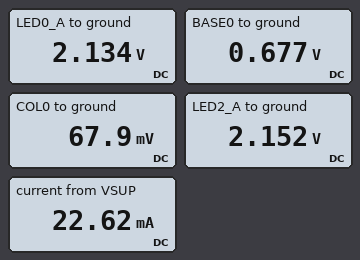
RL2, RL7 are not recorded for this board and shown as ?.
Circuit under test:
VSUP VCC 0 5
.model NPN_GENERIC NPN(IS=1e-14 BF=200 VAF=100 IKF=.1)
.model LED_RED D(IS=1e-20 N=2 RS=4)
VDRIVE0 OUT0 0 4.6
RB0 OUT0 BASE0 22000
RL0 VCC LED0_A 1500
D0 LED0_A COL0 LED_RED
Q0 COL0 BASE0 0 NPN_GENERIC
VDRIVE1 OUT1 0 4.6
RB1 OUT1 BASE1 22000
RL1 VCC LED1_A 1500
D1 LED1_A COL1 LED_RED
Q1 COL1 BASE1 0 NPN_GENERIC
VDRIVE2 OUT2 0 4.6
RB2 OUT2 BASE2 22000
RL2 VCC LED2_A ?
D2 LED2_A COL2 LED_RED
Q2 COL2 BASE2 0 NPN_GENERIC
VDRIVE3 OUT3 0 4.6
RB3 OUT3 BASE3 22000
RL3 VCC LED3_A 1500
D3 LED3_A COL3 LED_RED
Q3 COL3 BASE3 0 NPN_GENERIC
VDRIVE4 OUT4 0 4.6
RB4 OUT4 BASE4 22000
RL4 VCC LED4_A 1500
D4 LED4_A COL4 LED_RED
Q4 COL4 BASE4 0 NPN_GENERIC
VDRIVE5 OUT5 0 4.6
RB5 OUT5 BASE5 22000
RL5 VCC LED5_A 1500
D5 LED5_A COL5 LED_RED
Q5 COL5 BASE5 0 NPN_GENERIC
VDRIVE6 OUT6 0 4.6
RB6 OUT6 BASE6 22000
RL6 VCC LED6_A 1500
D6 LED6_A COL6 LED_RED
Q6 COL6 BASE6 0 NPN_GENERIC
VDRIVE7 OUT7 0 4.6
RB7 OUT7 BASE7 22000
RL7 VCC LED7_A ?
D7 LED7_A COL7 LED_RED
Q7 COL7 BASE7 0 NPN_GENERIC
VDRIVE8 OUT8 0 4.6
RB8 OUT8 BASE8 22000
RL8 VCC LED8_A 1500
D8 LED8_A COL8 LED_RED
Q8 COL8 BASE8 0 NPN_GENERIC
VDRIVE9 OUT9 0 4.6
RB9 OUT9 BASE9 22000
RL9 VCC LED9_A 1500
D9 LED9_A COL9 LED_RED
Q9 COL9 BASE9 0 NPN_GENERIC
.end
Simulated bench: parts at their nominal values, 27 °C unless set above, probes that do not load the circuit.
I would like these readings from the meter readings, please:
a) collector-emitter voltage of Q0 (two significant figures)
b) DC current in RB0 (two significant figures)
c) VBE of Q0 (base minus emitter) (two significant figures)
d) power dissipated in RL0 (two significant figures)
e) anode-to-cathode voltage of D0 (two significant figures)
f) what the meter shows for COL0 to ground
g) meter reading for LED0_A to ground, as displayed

68 mV
180 µA
680 mV
5.5 mW
2.1 V
67.9 mV
2.134 V
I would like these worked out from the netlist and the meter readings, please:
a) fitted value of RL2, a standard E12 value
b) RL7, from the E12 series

1.2 kΩ
560 Ω
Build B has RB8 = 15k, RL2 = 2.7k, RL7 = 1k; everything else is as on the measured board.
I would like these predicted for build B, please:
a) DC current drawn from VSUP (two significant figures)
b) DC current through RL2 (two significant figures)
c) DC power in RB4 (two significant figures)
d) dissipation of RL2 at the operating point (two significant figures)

19 mA
1.1 mA
700 µW
3.1 mW
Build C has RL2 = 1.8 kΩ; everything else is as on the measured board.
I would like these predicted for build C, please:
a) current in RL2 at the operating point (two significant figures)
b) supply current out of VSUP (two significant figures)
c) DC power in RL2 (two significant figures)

1.6 mA
22 mA
4.6 mW
